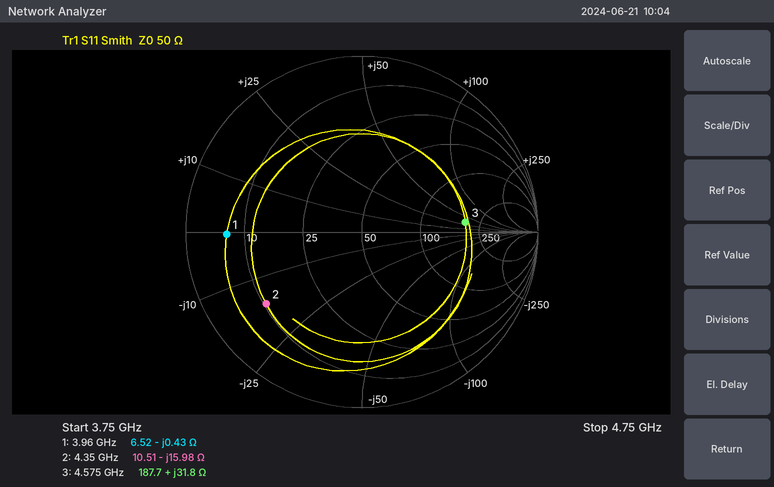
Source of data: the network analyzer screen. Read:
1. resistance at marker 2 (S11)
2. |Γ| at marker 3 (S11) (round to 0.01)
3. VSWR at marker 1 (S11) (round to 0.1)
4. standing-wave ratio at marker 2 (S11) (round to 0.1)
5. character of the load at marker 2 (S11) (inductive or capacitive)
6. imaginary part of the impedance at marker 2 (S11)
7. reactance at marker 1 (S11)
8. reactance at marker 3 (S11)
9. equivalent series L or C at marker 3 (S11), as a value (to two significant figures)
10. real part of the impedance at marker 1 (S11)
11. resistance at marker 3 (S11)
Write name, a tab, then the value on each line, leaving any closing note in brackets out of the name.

resistance at marker 2	10.51 Ω
|Γ| at marker 3 (S11)	0.59
VSWR at marker 1 (S11)	7.7
standing-wave ratio at marker 2 (S11)	5.3
character of the load at marker 2 (S11)	capacitive
imaginary part of the impedance at marker 2	-15.98 Ω
reactance at marker 1	-0.43 Ω
reactance at marker 3	+31.8 Ω
equivalent series L or C at marker 3 (S11), as a value	1.1 nH
real part of the impedance at marker 1	6.52 Ω
resistance at marker 3	187.7 Ω
